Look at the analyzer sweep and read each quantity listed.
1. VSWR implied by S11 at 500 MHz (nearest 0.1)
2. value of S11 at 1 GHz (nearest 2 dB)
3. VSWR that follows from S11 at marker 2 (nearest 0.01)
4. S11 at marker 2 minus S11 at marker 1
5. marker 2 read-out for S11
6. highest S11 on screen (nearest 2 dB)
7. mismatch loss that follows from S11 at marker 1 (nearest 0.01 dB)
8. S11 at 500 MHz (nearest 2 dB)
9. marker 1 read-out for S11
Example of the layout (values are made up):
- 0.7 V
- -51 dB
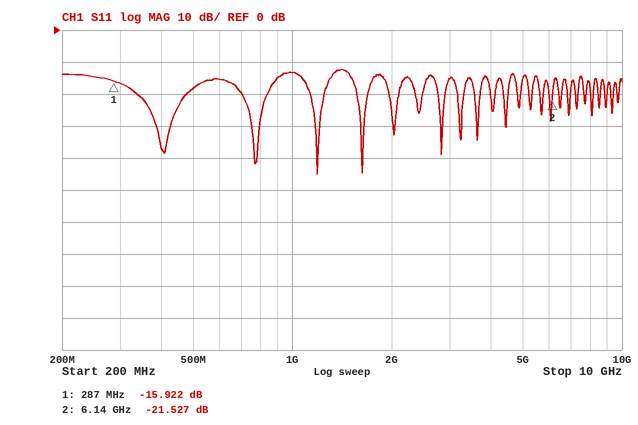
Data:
- 1.3
- -14 dB
- 1.18
- -5.605 dB
- -21.527 dB
- -12 dB
- 0.11 dB
- -18 dB
- -15.922 dB
